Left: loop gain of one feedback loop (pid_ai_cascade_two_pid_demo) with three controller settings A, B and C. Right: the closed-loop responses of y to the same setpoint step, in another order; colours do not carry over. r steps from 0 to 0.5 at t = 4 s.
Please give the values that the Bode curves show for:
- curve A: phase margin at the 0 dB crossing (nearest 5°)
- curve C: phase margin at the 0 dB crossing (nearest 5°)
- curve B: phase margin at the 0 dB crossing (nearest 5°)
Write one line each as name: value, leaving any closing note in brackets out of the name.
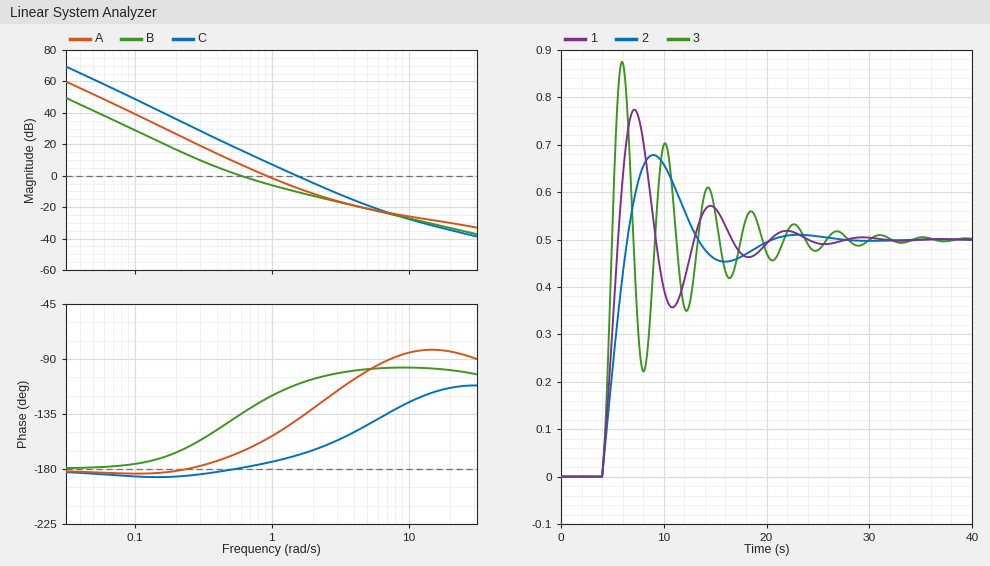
curve A: phase margin at the 0 dB crossing: 25°
curve C: phase margin at the 0 dB crossing: 10°
curve B: phase margin at the 0 dB crossing: 45°
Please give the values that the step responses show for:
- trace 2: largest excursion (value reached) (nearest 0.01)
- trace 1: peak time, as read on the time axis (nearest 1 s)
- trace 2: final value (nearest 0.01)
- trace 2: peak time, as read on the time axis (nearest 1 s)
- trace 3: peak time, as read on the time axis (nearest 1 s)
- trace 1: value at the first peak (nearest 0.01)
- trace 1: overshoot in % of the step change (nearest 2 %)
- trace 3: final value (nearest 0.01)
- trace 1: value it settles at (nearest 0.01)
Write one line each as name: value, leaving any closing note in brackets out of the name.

trace 2: largest excursion (value reached): 0.68
trace 1: peak time, as read on the time axis: 7 s
trace 2: final value: 0.50
trace 2: peak time, as read on the time axis: 9 s
trace 3: peak time, as read on the time axis: 6 s
trace 1: value at the first peak: 0.77
trace 1: overshoot in % of the step change: 54 %
trace 3: final value: 0.50
trace 1: value it settles at: 0.50
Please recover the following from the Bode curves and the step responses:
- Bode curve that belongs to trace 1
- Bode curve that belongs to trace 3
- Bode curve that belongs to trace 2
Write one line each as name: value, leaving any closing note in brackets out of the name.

Bode curve that belongs to trace 1: A
Bode curve that belongs to trace 3: C
Bode curve that belongs to trace 2: B
